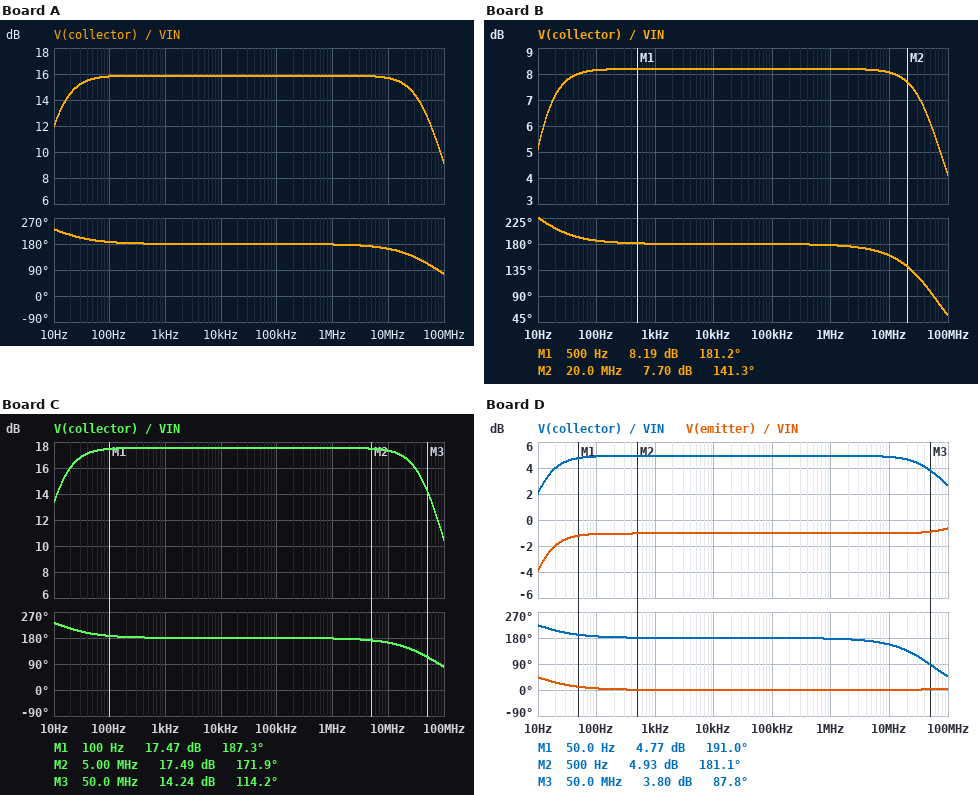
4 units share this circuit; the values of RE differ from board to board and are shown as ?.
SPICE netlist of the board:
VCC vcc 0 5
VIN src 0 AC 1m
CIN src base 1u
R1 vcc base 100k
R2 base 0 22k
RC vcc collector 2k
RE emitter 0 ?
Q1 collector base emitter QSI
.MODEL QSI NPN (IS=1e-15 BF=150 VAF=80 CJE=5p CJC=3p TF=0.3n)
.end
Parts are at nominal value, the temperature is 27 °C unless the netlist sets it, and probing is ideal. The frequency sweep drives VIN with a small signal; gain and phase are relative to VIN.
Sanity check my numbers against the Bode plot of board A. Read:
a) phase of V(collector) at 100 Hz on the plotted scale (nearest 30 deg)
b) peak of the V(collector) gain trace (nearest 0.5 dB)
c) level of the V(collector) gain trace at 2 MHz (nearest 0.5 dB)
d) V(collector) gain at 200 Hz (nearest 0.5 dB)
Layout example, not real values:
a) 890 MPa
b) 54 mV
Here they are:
a) 180 deg
b) 16.0 dB
c) 16.0 dB
d) 16.0 dB
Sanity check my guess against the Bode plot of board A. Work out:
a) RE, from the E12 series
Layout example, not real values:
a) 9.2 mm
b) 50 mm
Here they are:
a) 270 Ω
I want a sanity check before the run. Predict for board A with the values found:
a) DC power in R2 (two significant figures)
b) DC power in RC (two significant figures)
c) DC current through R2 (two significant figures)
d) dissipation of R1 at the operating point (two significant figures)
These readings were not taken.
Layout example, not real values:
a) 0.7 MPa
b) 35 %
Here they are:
a) 32 µW
b) 560 µW
c) 38 µA
d) 170 µW
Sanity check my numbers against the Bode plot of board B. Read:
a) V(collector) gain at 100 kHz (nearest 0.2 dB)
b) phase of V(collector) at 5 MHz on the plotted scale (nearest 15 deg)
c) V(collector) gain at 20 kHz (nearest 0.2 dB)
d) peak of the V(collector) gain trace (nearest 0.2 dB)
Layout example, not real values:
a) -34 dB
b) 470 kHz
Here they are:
a) 8.2 dB
b) 165 deg
c) 8.2 dB
d) 8.2 dB
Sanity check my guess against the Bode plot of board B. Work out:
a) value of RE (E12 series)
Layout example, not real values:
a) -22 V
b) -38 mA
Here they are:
a) 680 Ω
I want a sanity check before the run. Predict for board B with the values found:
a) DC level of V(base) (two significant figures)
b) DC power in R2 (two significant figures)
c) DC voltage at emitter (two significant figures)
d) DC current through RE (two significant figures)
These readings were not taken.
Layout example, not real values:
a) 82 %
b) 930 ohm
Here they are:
a) 870 mV
b) 34 µW
c) 190 mV
d) 280 µA
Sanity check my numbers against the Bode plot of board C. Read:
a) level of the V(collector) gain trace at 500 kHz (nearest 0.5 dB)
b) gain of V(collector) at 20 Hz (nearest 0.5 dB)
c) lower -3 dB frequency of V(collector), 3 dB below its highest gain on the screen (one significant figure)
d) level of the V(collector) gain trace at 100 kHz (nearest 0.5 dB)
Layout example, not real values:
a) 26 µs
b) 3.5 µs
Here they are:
a) 17.5 dB
b) 16.0 dB
c) 10 Hz
d) 17.5 dB
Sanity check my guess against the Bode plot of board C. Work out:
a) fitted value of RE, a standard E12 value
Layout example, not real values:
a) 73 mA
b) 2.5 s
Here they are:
a) 220 Ω
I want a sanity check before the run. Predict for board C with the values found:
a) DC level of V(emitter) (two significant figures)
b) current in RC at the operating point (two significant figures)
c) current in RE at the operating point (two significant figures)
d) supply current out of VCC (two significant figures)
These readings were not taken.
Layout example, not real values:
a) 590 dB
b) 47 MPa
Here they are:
a) 130 mV
b) 600 µA
c) 600 µA
d) 640 µA
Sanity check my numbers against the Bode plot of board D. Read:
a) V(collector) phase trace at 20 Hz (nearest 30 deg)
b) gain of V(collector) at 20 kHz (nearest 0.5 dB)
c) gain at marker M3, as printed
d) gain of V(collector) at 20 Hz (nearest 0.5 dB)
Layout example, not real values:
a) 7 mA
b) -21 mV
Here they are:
a) 210 deg
b) 5.0 dB
c) 3.80 dB
d) 4.0 dB
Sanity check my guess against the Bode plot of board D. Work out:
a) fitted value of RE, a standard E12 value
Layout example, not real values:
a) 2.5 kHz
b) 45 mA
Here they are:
a) 1 kΩ
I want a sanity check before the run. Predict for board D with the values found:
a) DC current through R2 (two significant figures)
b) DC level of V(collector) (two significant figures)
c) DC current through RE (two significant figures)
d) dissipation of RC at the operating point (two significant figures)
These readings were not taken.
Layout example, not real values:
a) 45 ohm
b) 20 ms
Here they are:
a) 40 µA
b) 4.6 V
c) 210 µA
d) 84 µW
